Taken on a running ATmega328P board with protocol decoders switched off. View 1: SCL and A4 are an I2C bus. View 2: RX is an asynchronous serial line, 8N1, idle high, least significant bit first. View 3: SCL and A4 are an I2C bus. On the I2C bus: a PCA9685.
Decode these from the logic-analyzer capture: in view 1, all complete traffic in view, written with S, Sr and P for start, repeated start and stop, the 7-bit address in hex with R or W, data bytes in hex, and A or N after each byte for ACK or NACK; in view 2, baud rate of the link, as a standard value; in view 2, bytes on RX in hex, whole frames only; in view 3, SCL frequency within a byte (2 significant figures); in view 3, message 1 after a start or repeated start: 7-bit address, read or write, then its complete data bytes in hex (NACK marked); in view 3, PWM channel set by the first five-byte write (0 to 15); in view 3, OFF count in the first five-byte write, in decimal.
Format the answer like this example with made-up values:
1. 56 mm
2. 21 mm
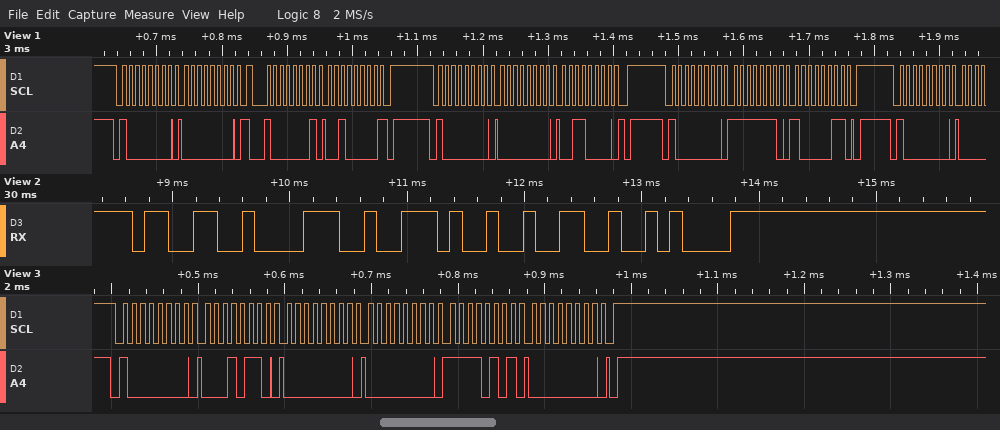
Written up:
1. S 40W A 00 A Sr 40R A 20 N P S 40W A 00 A 30 A P S 40W A FE A 83 A P S 40W A
2. 9600 baud
3. 33 38 2E 32 0A
4. 100 kHz
5. 0x40 write: 16 00 00 F5 00
6. 4
7. 245
